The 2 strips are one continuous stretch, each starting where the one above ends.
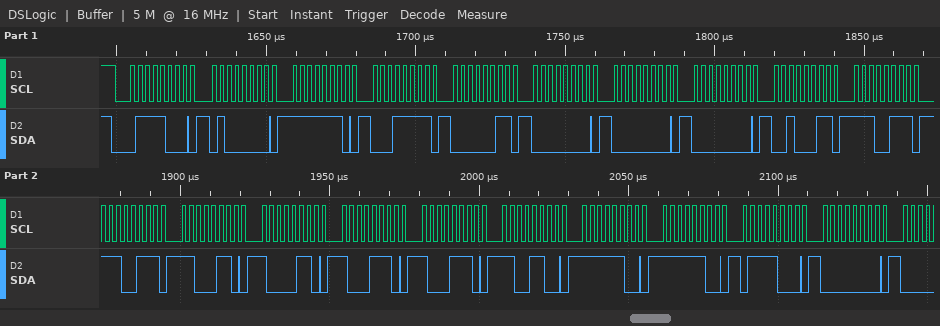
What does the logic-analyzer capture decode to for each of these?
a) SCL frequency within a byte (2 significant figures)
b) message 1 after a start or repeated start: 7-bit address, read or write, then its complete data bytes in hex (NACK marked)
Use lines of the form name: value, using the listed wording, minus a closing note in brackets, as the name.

SCL frequency within a byte: 400 kHz
message 1 after a start or repeated start: 7-bit address, read or write, then its complete data bytes in hex: 0x3C write: 40 FE 1F 03 00 00 00 23 E7 E7 C6 86 8E 8E CC FC FC 78 00
